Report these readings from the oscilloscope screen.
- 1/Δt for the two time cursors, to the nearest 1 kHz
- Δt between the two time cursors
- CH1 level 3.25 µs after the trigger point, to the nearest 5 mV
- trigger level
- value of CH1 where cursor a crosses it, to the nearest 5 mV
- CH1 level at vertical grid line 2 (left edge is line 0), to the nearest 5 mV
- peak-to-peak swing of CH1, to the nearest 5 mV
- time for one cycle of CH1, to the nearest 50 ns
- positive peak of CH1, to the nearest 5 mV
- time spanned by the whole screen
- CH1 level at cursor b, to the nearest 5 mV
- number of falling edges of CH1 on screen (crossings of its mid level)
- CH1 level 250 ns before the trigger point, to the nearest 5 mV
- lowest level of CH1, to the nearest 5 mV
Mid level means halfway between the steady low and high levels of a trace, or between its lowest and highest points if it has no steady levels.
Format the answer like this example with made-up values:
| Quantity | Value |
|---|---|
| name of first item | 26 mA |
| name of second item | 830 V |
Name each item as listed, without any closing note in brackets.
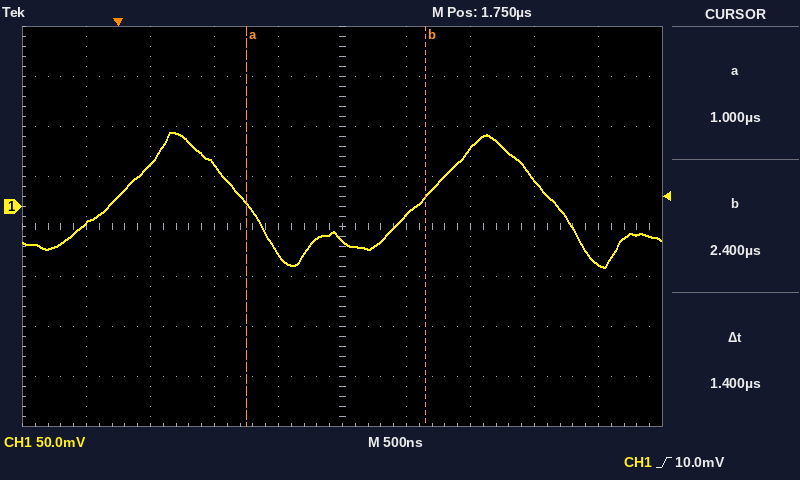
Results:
| Quantity | Value |
|---|---|
| 1/Δt for the two time cursors, to the nearest 1 kHz | 714 kHz |
| Δt between the two time cursors | 1.4 µs |
| CH1 level 3.25 µs after the trigger point, to the nearest 5 mV | 25 mV |
| trigger level | 10.0 mV |
| value of CH1 where cursor a crosses it, to the nearest 5 mV | 5 mV |
| CH1 level at vertical grid line 2 (left edge is line 0), to the nearest 5 mV | 40 mV |
| peak-to-peak swing of CH1, to the nearest 5 mV | 135 mV |
| time for one cycle of CH1, to the nearest 50 ns | 2.40 µs |
| positive peak of CH1, to the nearest 5 mV | 75 mV |
| time spanned by the whole screen | 5 µs |
| CH1 level at cursor b, to the nearest 5 mV | 10 mV |
| number of falling edges of CH1 on screen | 2 |
| CH1 level 250 ns before the trigger point, to the nearest 5 mV | -15 mV |
| lowest level of CH1, to the nearest 5 mV | -60 mV |
